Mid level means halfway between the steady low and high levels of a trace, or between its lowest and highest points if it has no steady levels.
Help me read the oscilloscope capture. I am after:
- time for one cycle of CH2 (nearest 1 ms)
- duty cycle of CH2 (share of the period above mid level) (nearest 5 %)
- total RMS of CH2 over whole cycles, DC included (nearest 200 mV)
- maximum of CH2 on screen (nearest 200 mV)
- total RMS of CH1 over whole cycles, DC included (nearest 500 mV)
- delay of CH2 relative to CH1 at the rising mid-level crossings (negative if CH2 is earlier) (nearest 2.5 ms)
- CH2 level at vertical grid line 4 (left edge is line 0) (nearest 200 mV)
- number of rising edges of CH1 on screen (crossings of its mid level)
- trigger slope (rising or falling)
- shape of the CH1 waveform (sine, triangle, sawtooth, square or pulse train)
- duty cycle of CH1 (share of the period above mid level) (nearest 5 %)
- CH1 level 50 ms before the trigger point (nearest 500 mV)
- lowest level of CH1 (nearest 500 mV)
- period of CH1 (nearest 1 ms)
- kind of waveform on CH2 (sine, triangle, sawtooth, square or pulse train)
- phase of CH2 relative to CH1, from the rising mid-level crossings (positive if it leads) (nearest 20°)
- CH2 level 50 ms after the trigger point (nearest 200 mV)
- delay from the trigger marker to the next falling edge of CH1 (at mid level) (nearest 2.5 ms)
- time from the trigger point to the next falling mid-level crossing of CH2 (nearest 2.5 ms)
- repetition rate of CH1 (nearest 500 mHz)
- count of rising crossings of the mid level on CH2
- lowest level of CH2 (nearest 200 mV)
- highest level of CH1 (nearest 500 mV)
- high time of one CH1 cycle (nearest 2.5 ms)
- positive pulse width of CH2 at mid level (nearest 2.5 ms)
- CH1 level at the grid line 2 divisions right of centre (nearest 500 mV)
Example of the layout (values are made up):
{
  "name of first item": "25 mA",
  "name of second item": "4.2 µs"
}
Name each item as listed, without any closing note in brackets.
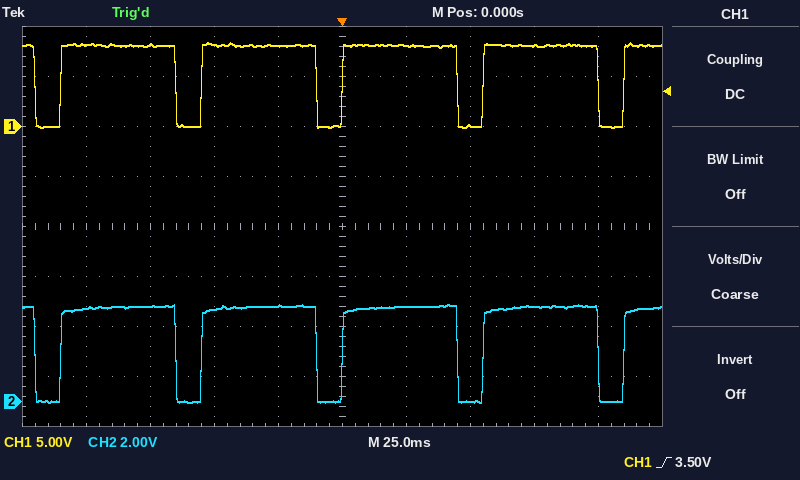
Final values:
{
  "time for one cycle of CH2": "55 ms",
  "duty cycle of CH2 (share of the period above mid level)": "80 %",
  "total RMS of CH2 over whole cycles, DC included": "3.4 V",
  "maximum of CH2 on screen": "3.8 V",
  "total RMS of CH1 over whole cycles, DC included": "7.5 V",
  "delay of CH2 relative to CH1 at the rising mid-level crossings (negative if CH2 is earlier)": "0.0 ms",
  "CH2 level at vertical grid line 4 (left edge is line 0)": "3.8 V",
  "number of rising edges of CH1 on screen": "5",
  "trigger slope": "rising",
  "shape of the CH1 waveform": "pulse train",
  "duty cycle of CH1 (share of the period above mid level)": "80 %",
  "CH1 level 50 ms before the trigger point": "8.0 V",
  "lowest level of CH1": "0.0 V",
  "period of CH1": "55 ms",
  "kind of waveform on CH2": "pulse train",
  "phase of CH2 relative to CH1, from the rising mid-level crossings (positive if it leads)": "0°",
  "CH2 level 50 ms after the trigger point": "0.0 V",
  "delay from the trigger marker to the next falling edge of CH1 (at mid level)": "45.0 ms",
  "time from the trigger point to the next falling mid-level crossing of CH2": "45.0 ms",
  "repetition rate of CH1": "18.0 Hz",
  "count of rising crossings of the mid level on CH2": "5",
  "lowest level of CH2": "0.0 V",
  "highest level of CH1": "8.5 V",
  "high time of one CH1 cycle": "45.0 ms",
  "positive pulse width of CH2 at mid level": "45.0 ms",
  "CH1 level at the grid line 2 divisions right of centre": "0.0 V"
}
